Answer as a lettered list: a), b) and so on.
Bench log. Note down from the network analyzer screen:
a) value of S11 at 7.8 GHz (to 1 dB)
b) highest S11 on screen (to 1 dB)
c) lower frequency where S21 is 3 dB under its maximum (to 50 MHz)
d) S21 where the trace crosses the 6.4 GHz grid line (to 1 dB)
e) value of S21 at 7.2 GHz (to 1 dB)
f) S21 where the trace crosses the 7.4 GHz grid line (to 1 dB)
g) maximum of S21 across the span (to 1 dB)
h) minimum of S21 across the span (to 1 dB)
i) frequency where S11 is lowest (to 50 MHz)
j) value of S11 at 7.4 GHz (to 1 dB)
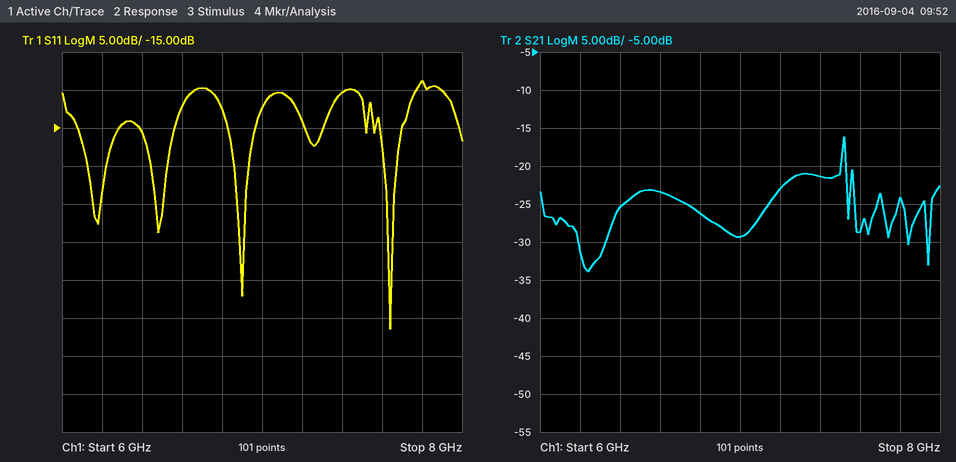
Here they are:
a) -9 dB
b) -9 dB
c) 7.50 GHz
d) -25 dB
e) -23 dB
f) -21 dB
g) -16 dB
h) -34 dB
i) 7.65 GHz
j) -10 dB
